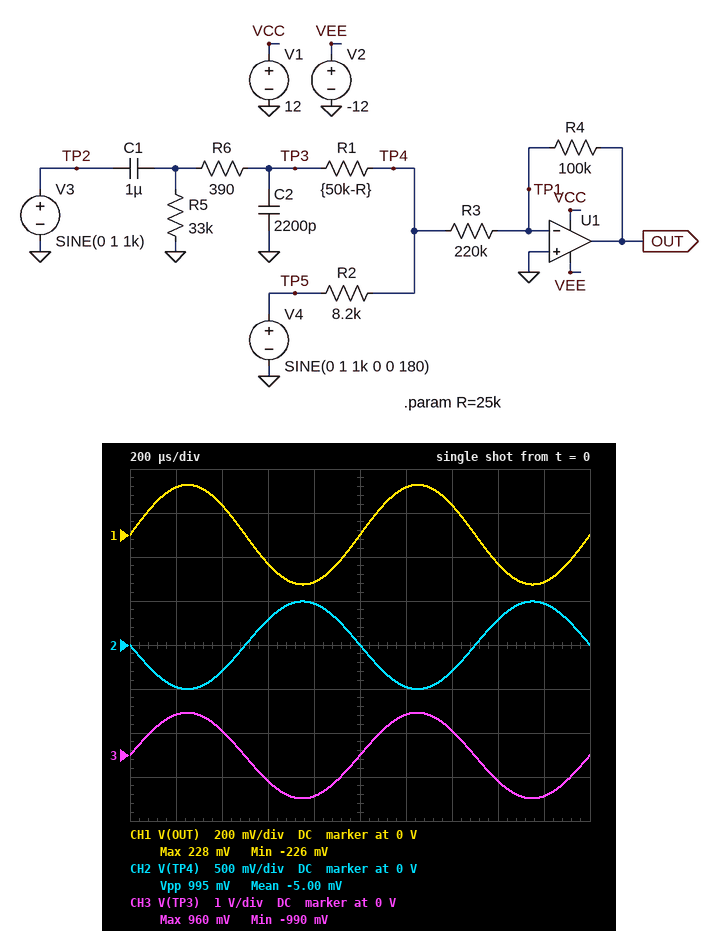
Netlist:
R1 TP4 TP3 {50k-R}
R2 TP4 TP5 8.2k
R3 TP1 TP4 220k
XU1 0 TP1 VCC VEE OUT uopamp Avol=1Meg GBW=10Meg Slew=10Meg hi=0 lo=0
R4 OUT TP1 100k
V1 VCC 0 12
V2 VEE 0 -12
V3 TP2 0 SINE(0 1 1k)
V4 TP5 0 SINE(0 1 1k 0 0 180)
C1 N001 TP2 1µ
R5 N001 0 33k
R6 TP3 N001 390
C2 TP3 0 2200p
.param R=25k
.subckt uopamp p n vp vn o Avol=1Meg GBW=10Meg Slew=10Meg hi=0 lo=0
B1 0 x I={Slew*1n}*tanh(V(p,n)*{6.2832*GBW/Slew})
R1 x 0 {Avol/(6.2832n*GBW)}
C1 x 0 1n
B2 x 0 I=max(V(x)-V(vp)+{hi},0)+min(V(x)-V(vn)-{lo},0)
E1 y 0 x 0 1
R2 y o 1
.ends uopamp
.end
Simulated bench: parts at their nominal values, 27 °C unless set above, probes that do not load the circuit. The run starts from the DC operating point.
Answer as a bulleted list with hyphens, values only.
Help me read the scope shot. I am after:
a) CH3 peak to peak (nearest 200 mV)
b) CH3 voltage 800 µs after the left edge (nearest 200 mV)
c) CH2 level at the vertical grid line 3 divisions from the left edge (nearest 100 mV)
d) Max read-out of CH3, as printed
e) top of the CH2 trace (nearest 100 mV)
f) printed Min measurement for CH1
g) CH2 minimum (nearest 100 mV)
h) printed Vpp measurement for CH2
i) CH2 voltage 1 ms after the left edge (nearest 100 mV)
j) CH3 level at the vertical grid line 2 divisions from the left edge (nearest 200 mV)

- 2.0 V
- -1.0 V
- 300 mV
- 960 mV
- 500 mV
- -226 mV
- -500 mV
- 995 mV
- 0 V
- 600 mV
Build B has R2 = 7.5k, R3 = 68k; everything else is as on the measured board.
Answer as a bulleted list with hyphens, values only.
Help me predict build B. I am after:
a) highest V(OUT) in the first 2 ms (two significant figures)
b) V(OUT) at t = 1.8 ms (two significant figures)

- 740 mV
- -700 mV
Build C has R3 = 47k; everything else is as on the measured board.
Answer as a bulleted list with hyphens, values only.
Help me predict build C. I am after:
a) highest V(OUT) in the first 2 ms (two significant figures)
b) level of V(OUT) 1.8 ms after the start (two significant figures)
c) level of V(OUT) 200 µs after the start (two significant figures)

- 970 mV
- -910 mV
- 920 mV
